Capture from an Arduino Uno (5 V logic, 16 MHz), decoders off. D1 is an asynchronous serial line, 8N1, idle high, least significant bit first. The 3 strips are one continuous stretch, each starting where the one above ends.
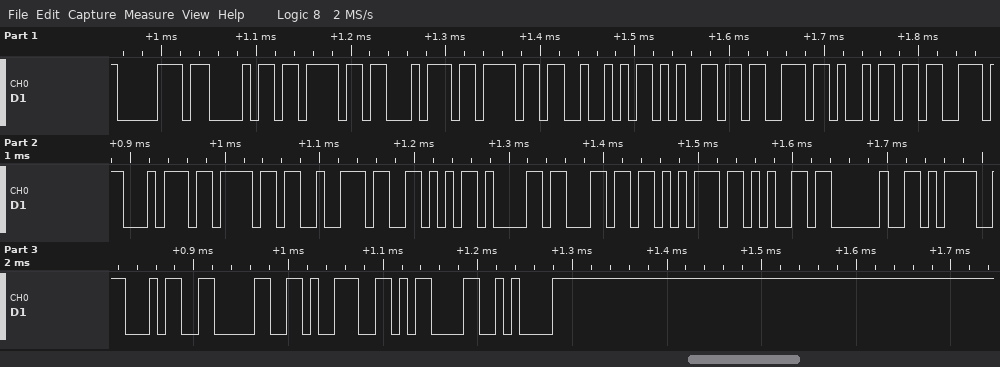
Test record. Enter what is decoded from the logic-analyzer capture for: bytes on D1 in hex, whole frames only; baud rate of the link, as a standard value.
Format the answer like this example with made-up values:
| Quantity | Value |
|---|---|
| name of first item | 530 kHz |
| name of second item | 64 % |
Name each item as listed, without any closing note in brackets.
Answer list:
| Quantity | Value |
|---|---|
| bytes on D1 in hex, whole frames only | 70 68 6F 74 6F 52 65 73 69 73 74 6F 72 56 61 6C 75 65 20 3D 34 30 39 0D 0A |
| baud rate of the link, as a standard value | 115200 baud |
